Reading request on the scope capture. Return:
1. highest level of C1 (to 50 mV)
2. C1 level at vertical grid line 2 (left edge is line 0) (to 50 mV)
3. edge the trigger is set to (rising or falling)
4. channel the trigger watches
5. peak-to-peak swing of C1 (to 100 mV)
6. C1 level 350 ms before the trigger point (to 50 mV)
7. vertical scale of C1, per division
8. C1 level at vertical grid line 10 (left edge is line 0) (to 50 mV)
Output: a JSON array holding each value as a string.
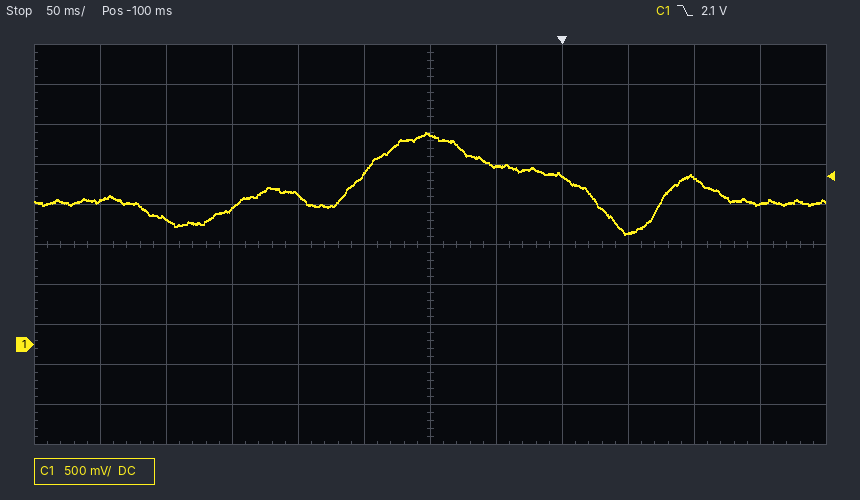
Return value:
["2.65 V", "1.55 V", "falling", "C1", "1.30 V", "1.80 V", "500 mV", "2.10 V"]
